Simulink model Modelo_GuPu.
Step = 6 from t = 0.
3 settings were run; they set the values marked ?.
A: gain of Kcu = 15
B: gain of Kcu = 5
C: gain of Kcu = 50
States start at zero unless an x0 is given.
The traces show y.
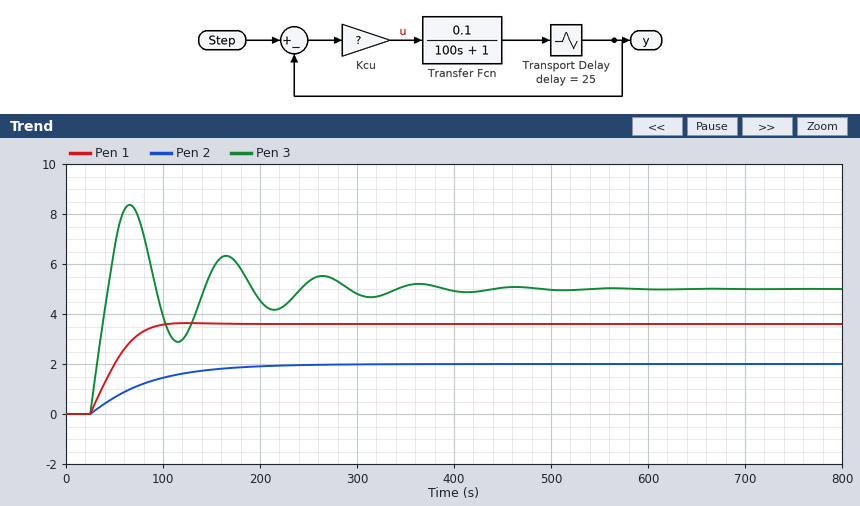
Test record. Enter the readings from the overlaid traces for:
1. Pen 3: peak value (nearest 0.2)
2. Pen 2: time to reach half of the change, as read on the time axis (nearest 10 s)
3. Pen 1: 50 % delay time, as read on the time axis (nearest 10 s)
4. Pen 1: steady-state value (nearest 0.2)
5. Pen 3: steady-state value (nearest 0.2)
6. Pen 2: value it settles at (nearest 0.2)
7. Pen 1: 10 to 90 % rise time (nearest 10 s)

8.4
70 s
50 s
3.6
5.0
2.0
50 s
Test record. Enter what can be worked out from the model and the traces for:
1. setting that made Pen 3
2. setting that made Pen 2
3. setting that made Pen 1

C
B
A
